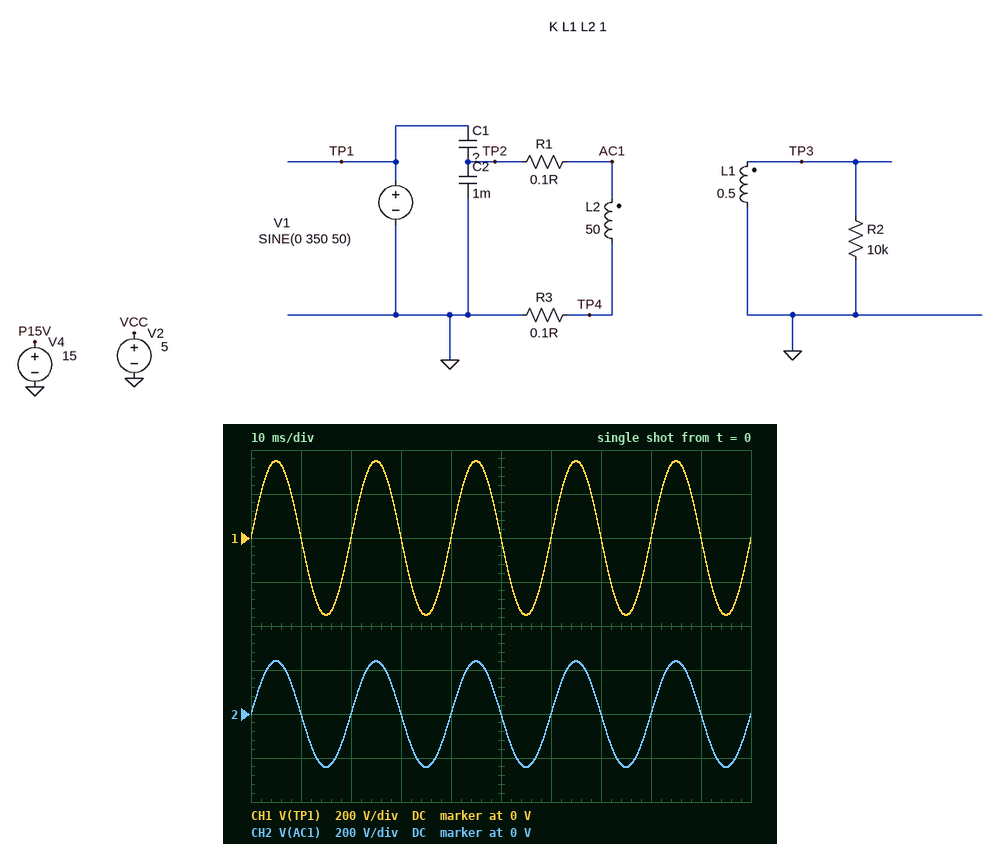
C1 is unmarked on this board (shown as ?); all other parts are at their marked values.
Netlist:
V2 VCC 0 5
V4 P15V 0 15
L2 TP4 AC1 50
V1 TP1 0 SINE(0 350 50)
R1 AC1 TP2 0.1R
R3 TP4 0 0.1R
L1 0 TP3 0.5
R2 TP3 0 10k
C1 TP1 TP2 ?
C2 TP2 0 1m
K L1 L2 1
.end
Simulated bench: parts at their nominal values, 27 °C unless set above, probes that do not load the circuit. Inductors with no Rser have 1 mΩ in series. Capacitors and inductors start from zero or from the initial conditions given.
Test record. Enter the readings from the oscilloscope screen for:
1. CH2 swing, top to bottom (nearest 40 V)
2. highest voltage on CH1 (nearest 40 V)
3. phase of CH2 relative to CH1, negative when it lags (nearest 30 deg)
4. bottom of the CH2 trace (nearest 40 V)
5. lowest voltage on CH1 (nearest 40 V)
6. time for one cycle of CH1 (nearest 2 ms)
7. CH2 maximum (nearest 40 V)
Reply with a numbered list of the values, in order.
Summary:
1. 480 V
2. 360 V
3. 0 deg
4. -240 V
5. -360 V
6. 20 ms
7. 240 V
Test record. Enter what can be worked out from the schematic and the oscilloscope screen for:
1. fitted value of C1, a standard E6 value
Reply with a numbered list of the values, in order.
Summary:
1. 2.2 mF
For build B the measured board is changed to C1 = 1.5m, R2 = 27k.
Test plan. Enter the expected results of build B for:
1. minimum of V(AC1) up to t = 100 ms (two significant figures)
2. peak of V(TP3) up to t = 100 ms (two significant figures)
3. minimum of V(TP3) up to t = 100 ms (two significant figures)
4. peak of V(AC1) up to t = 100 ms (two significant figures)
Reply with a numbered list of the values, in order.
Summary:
1. -210 V
2. 21 V
3. -21 V
4. 210 V
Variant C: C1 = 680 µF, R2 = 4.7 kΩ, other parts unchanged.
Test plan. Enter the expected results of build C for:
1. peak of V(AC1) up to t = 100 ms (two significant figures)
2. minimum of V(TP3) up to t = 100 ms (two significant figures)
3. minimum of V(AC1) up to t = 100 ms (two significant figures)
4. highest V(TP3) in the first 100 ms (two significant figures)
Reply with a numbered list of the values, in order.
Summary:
1. 140 V
2. -14 V
3. -140 V
4. 14 V
